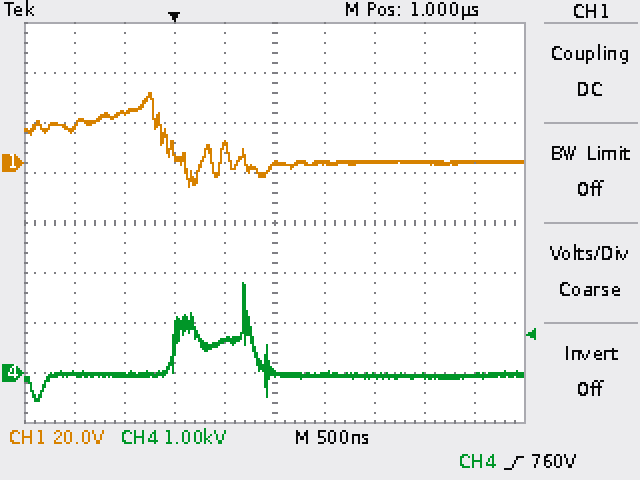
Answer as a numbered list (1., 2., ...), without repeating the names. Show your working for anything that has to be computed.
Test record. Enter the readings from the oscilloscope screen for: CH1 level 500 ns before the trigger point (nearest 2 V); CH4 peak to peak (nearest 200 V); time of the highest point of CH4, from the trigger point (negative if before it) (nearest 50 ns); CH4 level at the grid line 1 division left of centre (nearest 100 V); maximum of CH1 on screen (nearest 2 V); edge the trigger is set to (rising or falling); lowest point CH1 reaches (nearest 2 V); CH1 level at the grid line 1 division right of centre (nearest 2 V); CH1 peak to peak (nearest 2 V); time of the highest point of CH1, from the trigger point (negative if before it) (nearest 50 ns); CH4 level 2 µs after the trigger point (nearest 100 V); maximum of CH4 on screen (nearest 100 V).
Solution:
1. 20 V
2. 2.4 kV
3. +700 ns
4. 700 V
5. 28 V
6. rising
7. -10 V
8. 0 V
9. 28 V − (-10 V) = 38 V
10. -250 ns
11. -100 V
12. 1.8 kV
